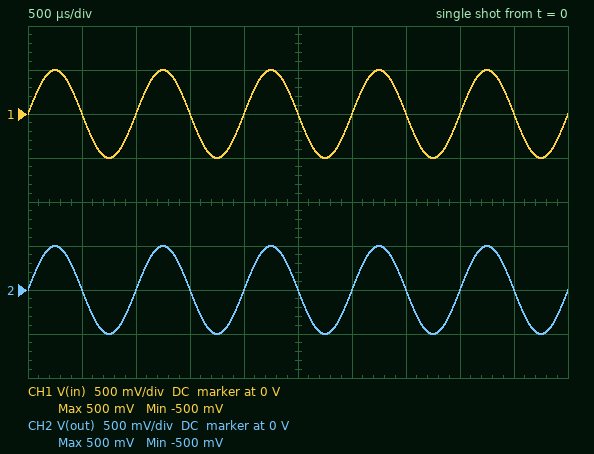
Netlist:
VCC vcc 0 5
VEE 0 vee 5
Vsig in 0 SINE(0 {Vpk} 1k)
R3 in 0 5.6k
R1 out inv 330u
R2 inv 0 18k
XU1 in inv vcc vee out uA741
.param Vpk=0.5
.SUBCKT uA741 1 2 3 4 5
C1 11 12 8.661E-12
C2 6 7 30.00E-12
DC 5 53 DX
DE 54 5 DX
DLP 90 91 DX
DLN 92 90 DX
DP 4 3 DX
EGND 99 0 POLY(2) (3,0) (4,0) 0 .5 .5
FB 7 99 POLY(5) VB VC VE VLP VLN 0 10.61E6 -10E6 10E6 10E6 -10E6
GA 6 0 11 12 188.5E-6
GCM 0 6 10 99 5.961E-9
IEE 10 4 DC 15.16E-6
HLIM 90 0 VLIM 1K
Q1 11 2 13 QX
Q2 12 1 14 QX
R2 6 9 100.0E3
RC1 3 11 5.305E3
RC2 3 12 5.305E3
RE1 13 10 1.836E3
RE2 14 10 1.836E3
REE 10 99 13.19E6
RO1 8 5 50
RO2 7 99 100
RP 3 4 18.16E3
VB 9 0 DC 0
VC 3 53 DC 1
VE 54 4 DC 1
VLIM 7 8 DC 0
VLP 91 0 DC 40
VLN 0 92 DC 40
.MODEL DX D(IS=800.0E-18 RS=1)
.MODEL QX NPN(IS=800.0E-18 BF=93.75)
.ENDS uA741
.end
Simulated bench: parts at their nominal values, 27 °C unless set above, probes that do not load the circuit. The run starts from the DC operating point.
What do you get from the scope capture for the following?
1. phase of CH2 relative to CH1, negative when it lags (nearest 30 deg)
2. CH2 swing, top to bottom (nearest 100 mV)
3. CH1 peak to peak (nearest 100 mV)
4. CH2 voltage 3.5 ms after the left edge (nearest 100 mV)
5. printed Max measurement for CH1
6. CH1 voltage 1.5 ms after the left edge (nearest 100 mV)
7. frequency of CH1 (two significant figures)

0 deg
1.0 V
1.0 V
0 V
500 mV
0 V
1.0 kHz
